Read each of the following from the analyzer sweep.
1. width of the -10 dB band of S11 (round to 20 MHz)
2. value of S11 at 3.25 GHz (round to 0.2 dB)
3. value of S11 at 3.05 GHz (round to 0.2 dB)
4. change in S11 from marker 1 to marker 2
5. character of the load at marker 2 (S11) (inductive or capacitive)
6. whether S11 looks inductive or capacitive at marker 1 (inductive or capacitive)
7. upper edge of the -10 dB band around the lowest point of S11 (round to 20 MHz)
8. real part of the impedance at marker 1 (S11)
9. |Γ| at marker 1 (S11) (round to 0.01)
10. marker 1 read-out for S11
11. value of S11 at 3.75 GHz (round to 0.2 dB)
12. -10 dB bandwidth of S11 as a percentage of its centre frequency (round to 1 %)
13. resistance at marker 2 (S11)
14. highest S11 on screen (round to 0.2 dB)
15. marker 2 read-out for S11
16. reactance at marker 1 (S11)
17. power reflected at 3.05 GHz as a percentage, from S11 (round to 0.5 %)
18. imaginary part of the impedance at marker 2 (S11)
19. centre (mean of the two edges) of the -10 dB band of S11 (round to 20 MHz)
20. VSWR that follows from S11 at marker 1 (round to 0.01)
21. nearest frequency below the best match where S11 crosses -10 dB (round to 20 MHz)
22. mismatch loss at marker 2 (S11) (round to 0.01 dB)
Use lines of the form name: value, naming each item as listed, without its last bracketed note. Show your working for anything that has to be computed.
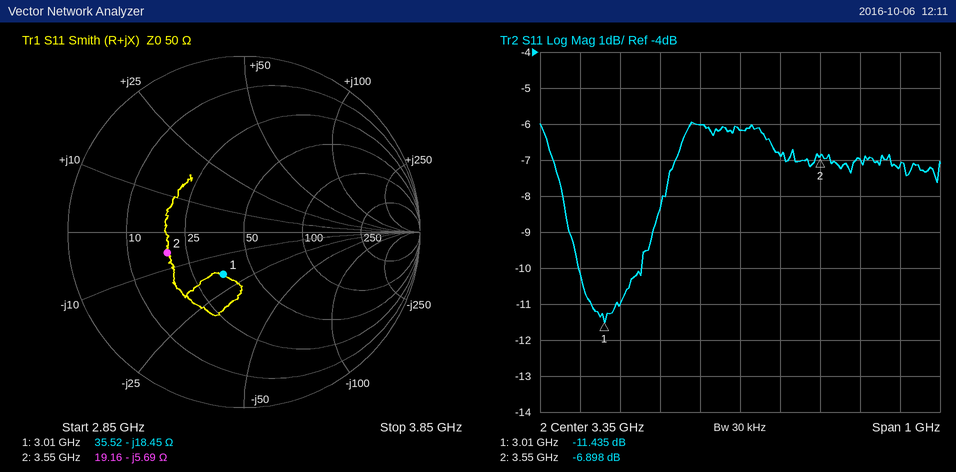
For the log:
width of the -10 dB band of S11: 3.10 GHz − 2.94 GHz = 160 MHz
value of S11 at 3.25 GHz: -6.0 dB
value of S11 at 3.05 GHz: -11.0 dB
change in S11 from marker 1 to marker 2: -6.898 − (-11.435) = 4.537 dB
character of the load at marker 2 (S11): capacitive
whether S11 looks inductive or capacitive at marker 1: capacitive
upper edge of the -10 dB band around the lowest point of S11: 3.10 GHz
real part of the impedance at marker 1: 35.52 Ω
|Γ| at marker 1 (S11): 0.27
marker 1 read-out for S11: -11.435 dB
value of S11 at 3.75 GHz: -7.2 dB
-10 dB bandwidth of S11 as a percentage of its centre frequency: 160 MHz / 3.02 GHz ≈ 5 %
resistance at marker 2: 19.16 Ω
highest S11 on screen: -6.0 dB
marker 2 read-out for S11: -6.898 dB
reactance at marker 1: -18.45 Ω
power reflected at 3.05 GHz as a percentage, from S11: 10^(-11/10) ≈ 7.94 %, so 8.0 % to the nearest 0.5 %
imaginary part of the impedance at marker 2: -5.69 Ω
centre (mean of the two edges) of the -10 dB band of S11: 3.02 GHz
VSWR that follows from S11 at marker 1: (1 + 0.2681)/(1 − 0.2681) ≈ 1.73
nearest frequency below the best match where S11 crosses -10 dB: 2.94 GHz
mismatch loss at marker 2 (S11): −10 log10(1 − 10^(-6.898/10)) ≈ 0.99 dB
